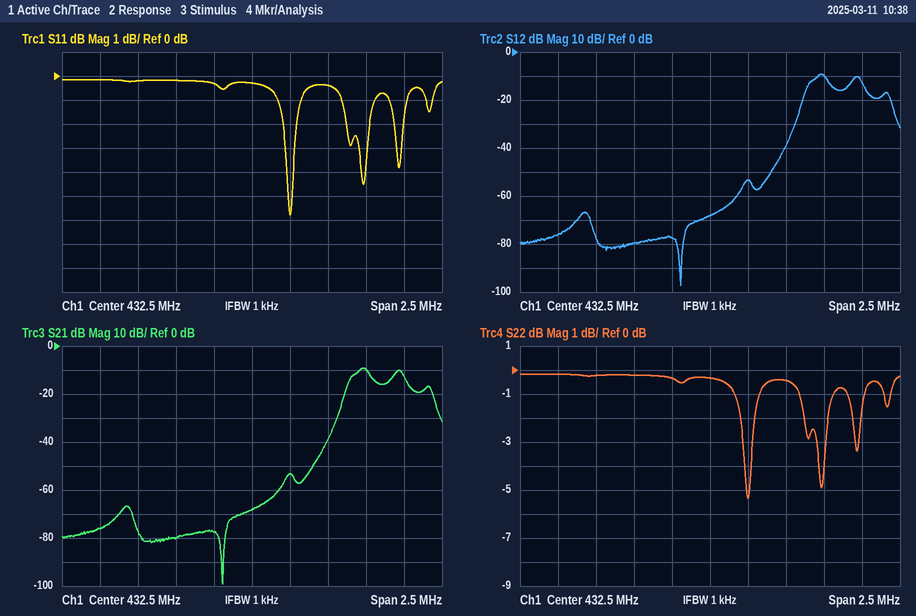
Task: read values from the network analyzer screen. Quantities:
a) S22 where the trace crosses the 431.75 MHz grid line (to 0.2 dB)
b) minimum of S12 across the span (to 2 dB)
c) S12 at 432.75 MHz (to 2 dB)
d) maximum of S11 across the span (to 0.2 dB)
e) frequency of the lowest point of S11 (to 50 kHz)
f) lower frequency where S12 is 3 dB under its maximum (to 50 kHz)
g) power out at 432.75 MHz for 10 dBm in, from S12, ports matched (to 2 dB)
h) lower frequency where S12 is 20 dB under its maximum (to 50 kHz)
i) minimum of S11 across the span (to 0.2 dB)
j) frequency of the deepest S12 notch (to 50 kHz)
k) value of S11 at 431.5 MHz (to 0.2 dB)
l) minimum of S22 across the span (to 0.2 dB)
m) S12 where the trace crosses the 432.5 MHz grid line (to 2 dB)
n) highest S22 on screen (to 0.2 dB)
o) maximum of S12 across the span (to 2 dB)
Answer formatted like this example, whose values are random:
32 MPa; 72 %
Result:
-0.2 dB; -98 dB; -54 dB; -0.2 dB; 432.75 MHz; 433.15 MHz; -44 dBm; 433.05 MHz; -5.8 dB; 432.30 MHz; -0.2 dB; -5.4 dB; -68 dB; -0.2 dB; -10 dB
